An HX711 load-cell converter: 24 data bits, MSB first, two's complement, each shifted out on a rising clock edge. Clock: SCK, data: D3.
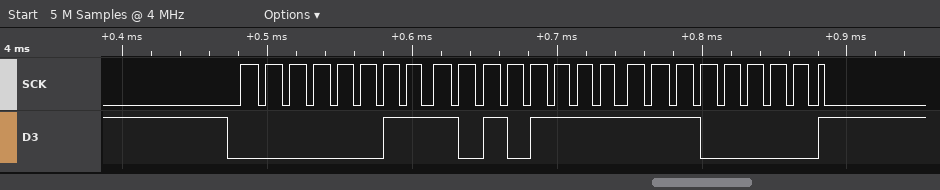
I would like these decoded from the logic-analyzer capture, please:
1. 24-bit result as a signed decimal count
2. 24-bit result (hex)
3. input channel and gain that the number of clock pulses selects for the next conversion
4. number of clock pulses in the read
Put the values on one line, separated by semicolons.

241632; 0x03AFE0; channel A, gain 128; 25
